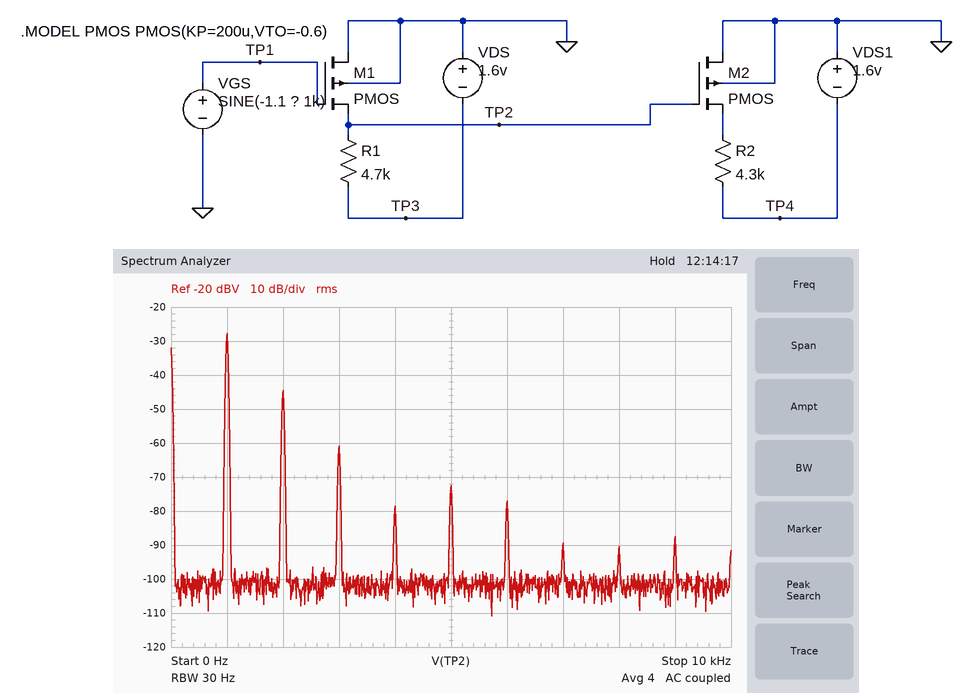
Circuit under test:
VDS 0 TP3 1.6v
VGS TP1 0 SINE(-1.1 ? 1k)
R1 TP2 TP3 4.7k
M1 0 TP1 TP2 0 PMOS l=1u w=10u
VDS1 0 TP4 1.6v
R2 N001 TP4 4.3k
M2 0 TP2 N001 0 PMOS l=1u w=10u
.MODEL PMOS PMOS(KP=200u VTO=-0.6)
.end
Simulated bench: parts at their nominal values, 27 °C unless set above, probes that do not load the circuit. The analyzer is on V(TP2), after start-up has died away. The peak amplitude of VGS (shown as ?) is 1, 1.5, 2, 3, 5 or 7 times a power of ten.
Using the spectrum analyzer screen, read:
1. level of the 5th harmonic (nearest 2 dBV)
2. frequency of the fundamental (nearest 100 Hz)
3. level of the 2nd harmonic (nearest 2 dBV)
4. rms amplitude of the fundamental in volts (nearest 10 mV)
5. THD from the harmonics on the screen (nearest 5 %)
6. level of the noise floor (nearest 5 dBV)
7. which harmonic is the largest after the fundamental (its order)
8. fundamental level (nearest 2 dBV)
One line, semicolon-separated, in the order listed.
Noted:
-72 dBV; 1.0 kHz; -44 dBV; 40 mV; 15 %; -100 dBV; 2; -28 dBV
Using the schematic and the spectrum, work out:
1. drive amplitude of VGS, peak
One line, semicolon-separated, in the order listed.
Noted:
20 mV
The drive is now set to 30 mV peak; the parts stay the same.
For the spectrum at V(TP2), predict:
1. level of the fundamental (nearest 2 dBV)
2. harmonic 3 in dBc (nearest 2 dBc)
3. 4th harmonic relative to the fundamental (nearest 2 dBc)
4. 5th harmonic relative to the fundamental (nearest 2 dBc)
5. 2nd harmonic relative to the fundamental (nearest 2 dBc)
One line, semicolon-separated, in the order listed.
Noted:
-24 dBV; -38 dBc; -36 dBc; -40 dBc; -16 dBc
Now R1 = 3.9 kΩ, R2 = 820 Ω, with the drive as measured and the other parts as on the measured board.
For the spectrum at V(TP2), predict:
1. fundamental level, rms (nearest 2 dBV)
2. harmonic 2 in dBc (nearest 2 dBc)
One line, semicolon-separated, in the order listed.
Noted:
-26 dBV; -40 dBc
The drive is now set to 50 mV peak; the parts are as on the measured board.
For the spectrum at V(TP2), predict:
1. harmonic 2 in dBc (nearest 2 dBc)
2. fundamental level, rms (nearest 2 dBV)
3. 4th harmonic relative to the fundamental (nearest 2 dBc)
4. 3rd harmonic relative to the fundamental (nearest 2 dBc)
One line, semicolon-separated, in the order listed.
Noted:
-14 dBc; -20 dBV; -30 dBc; -46 dBc
